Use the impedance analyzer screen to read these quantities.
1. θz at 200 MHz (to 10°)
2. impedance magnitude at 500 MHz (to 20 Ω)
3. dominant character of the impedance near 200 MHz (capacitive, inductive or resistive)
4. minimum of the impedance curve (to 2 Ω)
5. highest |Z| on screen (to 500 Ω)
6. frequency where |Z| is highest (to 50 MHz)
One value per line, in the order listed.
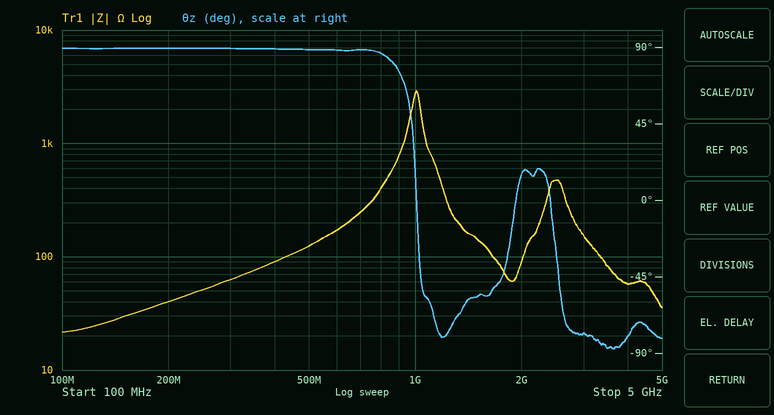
90°
120 Ω
inductive
22 Ω
3.0 kΩ
1.00 GHz
